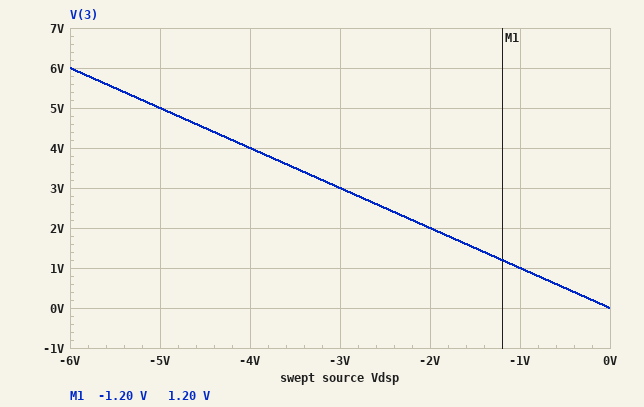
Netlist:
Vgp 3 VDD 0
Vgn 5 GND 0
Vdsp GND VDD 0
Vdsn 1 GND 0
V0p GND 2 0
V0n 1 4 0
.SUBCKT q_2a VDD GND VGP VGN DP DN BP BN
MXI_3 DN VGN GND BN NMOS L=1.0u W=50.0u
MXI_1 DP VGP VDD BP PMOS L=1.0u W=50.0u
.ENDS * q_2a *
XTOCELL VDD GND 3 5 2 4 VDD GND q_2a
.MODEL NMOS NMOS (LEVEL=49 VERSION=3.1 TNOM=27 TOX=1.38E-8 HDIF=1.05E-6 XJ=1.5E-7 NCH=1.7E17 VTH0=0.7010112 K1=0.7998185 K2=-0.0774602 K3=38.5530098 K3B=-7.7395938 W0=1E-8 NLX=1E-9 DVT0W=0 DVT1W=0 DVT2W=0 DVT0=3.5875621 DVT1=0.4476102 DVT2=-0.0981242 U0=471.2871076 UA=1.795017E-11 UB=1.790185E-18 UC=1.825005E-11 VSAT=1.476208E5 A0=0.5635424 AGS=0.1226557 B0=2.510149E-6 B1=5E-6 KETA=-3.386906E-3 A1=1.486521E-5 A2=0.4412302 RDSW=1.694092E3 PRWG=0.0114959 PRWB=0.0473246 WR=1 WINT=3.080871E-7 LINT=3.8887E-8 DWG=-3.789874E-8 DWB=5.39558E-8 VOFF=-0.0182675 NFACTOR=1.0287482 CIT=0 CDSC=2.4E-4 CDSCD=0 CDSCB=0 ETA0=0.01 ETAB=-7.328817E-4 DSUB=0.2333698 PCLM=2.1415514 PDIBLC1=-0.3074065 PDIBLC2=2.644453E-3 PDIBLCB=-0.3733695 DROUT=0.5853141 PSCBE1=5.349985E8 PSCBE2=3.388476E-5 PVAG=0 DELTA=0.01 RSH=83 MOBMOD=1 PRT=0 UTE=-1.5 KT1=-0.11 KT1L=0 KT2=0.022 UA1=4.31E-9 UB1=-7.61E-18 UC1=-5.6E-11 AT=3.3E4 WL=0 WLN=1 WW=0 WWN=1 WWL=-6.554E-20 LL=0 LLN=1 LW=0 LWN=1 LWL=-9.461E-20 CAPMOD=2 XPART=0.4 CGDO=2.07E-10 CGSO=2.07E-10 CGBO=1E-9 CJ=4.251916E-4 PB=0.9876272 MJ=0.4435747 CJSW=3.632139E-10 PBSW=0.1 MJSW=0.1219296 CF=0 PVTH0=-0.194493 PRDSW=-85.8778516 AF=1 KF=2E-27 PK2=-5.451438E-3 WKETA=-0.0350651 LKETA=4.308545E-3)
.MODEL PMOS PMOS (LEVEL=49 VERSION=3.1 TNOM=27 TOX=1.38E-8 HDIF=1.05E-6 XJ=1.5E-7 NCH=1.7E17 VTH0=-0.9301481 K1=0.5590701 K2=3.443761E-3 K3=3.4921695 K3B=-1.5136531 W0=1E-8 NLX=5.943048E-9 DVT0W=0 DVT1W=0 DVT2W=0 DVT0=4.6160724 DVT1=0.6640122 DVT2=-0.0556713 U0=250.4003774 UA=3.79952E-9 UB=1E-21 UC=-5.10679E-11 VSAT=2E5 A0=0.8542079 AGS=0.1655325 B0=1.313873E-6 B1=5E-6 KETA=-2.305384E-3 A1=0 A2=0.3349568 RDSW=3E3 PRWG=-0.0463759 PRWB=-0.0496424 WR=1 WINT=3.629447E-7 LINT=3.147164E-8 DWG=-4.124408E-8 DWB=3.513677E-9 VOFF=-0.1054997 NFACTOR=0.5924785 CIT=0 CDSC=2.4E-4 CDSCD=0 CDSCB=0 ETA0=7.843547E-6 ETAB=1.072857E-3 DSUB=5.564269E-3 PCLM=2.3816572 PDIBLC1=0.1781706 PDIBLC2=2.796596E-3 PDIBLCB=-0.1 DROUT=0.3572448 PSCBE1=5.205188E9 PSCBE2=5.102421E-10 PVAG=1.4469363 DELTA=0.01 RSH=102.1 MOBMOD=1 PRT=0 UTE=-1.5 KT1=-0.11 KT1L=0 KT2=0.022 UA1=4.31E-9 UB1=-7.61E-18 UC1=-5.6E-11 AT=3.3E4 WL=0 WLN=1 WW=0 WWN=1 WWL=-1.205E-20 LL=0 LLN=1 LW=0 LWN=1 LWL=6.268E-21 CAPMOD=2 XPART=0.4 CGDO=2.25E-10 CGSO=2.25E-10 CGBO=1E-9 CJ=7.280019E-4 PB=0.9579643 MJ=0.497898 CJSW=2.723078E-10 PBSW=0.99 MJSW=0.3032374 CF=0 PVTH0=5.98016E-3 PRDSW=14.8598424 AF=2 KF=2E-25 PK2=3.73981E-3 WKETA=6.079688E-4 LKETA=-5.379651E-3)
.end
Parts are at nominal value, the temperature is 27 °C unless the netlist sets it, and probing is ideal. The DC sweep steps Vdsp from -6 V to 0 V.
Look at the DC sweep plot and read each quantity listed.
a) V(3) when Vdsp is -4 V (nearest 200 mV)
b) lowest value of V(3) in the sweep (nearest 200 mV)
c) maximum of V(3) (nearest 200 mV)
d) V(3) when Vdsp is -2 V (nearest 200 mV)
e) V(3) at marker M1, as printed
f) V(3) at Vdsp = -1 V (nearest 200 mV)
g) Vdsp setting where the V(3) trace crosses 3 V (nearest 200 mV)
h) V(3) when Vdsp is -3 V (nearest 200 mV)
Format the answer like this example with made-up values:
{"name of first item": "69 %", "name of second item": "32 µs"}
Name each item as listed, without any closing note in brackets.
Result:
{"V(3) when Vdsp is -4 V": "4.0 V", "lowest value of V(3) in the sweep": "0 V", "maximum of V(3)": "6.0 V", "V(3) when Vdsp is -2 V": "2.0 V", "V(3) at marker M1, as printed": "1.20 V", "V(3) at Vdsp = -1 V": "1.0 V", "Vdsp setting where the V(3) trace crosses 3 V": "-3.0 V", "V(3) when Vdsp is -3 V": "3.0 V"}
